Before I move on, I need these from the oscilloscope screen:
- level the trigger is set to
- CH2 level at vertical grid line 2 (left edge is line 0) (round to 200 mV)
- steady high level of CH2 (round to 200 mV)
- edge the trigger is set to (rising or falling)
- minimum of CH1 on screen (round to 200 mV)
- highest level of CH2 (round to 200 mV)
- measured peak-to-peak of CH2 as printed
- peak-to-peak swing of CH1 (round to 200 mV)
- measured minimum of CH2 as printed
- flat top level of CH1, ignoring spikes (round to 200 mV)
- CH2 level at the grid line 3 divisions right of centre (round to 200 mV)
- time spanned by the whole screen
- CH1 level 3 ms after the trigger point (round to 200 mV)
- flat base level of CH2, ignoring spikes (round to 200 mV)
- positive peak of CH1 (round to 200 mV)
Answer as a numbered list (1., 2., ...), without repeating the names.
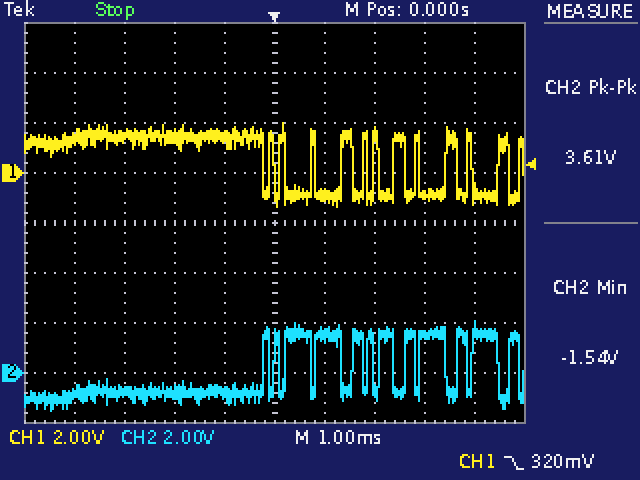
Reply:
1. 320 mV
2. -800 mV
3. 1.6 V
4. falling
5. -1.4 V
6. 2.0 V
7. 3.61 V
8. 3.4 V
9. -1.54 V
10. 1.4 V
11. 1.6 V
12. 10 ms
13. -800 mV
14. -800 mV
15. 2.0 V
